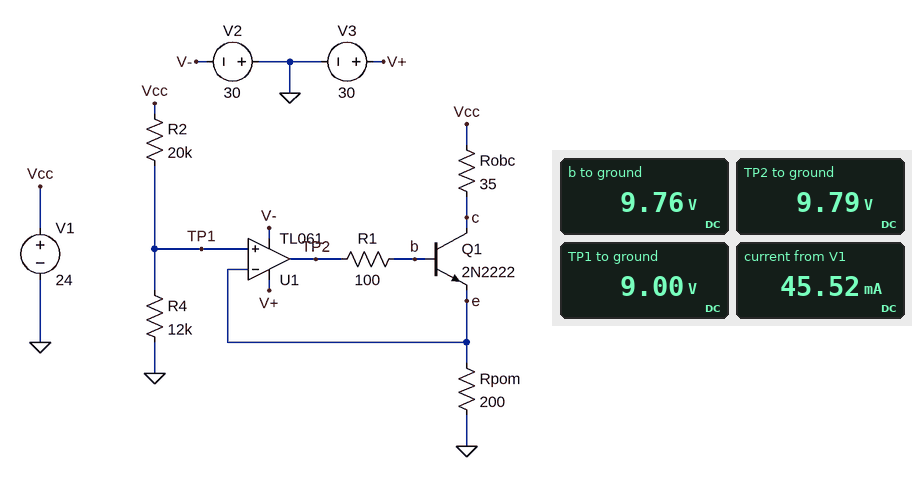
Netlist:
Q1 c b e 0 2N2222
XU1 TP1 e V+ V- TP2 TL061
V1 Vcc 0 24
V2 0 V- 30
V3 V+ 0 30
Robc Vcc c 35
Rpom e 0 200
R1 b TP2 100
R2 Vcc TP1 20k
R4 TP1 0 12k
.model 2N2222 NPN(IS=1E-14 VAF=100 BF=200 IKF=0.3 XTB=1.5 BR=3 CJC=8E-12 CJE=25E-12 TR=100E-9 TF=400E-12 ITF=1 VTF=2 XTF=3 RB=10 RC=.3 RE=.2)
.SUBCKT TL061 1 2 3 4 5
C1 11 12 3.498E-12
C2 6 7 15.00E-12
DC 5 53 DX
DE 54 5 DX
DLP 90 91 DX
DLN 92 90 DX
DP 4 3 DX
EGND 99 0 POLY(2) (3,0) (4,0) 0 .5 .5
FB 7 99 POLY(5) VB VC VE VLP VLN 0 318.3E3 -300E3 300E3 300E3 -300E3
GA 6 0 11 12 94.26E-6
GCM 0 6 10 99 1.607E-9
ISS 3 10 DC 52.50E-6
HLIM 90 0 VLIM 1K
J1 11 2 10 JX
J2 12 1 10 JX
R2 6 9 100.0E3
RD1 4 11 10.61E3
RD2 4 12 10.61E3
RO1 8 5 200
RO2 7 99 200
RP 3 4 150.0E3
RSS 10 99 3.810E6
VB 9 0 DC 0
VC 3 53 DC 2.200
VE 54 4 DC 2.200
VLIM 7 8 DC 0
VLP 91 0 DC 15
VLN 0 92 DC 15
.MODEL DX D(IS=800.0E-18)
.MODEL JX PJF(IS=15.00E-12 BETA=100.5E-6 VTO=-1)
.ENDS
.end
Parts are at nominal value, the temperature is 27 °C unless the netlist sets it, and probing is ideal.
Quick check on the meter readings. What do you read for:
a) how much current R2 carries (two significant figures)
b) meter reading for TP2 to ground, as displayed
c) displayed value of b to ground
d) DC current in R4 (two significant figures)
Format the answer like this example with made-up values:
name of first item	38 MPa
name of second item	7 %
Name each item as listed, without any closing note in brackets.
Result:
how much current R2 carries	750 µA
meter reading for TP2 to ground, as displayed	9.79 V
displayed value of b to ground	9.76 V
DC current in R4	750 µA
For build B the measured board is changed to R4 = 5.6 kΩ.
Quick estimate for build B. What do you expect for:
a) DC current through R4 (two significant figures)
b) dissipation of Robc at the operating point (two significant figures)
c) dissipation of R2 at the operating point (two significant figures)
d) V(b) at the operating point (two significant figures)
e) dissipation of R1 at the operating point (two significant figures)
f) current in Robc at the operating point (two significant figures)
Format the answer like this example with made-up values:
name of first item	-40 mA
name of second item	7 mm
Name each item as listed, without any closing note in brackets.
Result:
DC current through R4	940 µA
dissipation of Robc at the operating point	24 mW
dissipation of R2 at the operating point	18 mW
V(b) at the operating point	6.0 V
dissipation of R1 at the operating point	1.4 µW
current in Robc at the operating point	26 mA
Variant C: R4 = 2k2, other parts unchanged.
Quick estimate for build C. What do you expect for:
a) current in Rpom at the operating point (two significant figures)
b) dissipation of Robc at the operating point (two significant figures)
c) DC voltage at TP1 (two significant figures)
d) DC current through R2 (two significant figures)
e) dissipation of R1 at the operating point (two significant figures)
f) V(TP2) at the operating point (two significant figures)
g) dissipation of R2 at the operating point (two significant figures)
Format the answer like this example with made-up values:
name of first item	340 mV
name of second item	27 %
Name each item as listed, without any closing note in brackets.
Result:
current in Rpom at the operating point	12 mA
dissipation of Robc at the operating point	4.9 mW
DC voltage at TP1	2.4 V
DC current through R2	1.1 mA
dissipation of R1 at the operating point	260 nW
V(TP2) at the operating point	3.1 V
dissipation of R2 at the operating point	23 mW
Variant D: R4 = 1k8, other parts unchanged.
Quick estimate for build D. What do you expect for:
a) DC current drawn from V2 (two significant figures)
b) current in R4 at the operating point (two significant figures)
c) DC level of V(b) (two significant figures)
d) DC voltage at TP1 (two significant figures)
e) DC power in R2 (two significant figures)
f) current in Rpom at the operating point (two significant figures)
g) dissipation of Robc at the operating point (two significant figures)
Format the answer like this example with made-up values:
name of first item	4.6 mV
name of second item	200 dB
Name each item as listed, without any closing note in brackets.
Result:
DC current drawn from V2	450 µA
current in R4 at the operating point	1.1 mA
DC level of V(b)	2.7 V
DC voltage at TP1	2.0 V
DC power in R2	24 mW
current in Rpom at the operating point	9.9 mA
dissipation of Robc at the operating point	3.4 mW
